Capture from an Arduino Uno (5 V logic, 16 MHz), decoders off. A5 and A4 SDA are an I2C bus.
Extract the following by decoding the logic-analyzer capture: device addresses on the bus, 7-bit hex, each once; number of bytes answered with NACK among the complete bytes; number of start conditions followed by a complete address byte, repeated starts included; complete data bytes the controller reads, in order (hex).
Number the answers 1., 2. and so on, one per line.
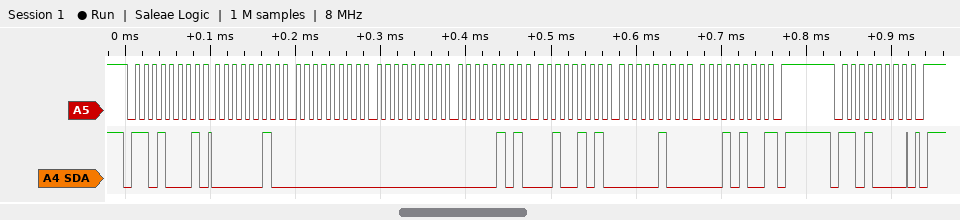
1. 0x68
2. 1
3. 2
4. 02 00 00 05 25 04 14
